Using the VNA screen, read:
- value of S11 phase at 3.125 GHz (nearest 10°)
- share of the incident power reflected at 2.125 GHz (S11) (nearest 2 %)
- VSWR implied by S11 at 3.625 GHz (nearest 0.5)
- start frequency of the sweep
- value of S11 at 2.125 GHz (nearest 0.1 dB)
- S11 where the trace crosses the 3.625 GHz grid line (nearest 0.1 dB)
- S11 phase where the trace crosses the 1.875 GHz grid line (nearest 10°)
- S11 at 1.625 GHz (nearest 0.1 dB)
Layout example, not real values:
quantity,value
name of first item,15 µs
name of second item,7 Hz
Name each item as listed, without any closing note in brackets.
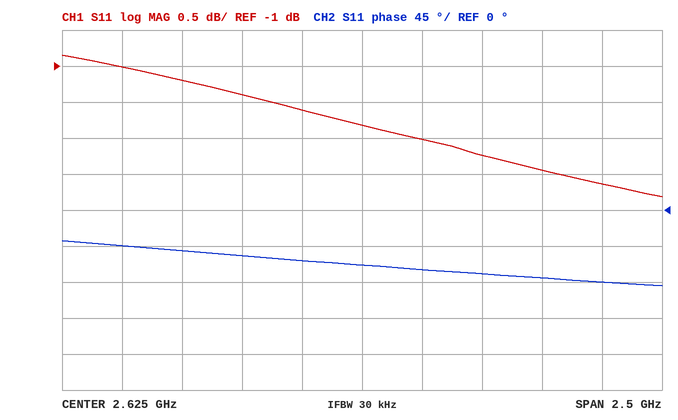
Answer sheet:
quantity,value
value of S11 phase at 3.125 GHz,-80°
share of the incident power reflected at 2.125 GHz (S11),72 %
VSWR implied by S11 at 3.625 GHz,6.5
start frequency of the sweep,1.375 GHz
value of S11 at 2.125 GHz,-1.4 dB
S11 where the trace crosses the 3.625 GHz grid line,-2.6 dB
S11 phase where the trace crosses the 1.875 GHz grid line,-50°
S11 at 1.625 GHz,-1.0 dB
